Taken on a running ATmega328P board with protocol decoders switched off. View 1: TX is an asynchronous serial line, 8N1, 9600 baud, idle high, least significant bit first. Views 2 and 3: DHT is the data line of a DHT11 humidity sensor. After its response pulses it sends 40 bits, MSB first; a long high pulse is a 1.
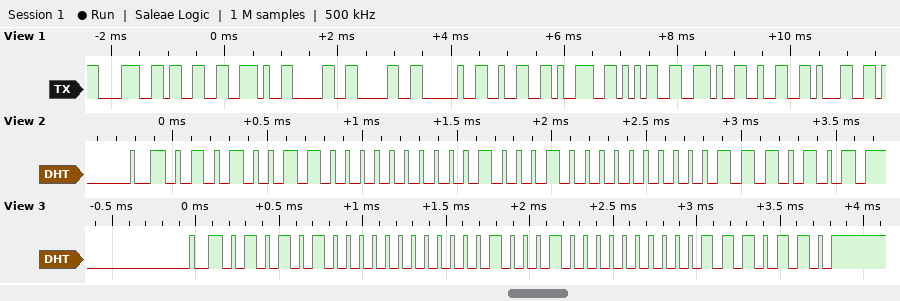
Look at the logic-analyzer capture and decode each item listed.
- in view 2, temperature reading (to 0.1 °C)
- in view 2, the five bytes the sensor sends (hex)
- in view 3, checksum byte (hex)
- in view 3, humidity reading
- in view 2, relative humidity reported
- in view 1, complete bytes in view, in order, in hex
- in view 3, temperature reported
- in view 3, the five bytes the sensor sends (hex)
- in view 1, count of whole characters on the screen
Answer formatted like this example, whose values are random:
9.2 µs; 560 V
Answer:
34.0 °C; 53 00 22 00 75; 0x76; 84 %; 83 %; 38 33 2E 30 30 20 32 39 35 2E 32 31; 34.0 °C; 54 00 22 00 76; 12
